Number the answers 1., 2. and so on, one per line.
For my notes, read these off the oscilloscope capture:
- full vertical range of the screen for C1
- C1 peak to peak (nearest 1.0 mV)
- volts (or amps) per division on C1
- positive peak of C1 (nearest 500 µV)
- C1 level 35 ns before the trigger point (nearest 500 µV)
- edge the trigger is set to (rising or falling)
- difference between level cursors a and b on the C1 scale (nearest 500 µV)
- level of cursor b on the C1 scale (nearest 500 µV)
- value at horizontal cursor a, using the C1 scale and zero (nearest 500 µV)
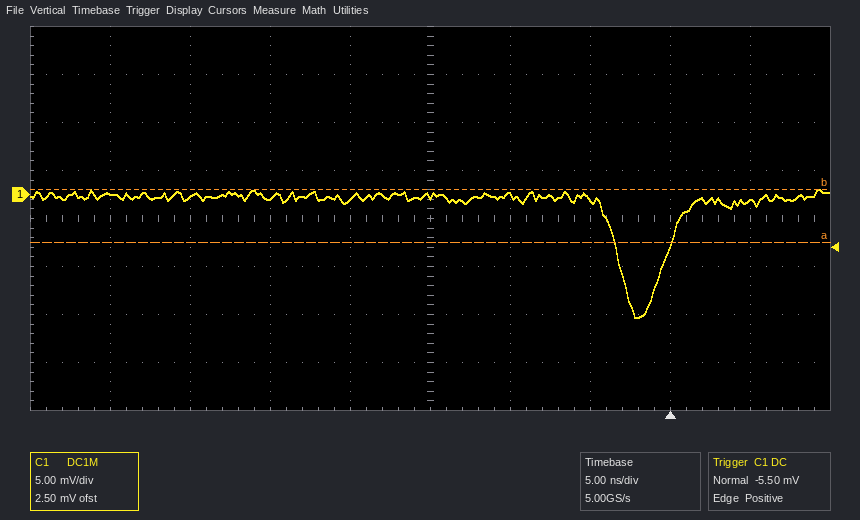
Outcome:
1. 40 mV
2. 13.0 mV
3. 5 mV
4. 500 µV
5. 0.0 mV
6. rising
7. 5.5 mV
8. 500 µV
9. -5.0 mV
